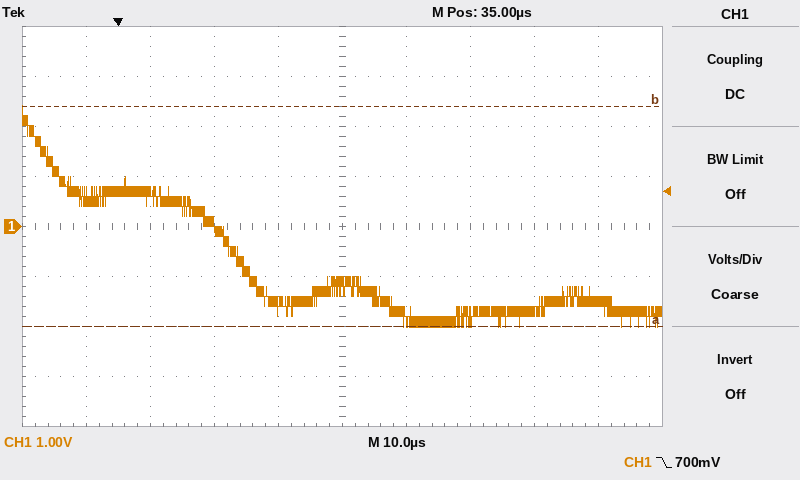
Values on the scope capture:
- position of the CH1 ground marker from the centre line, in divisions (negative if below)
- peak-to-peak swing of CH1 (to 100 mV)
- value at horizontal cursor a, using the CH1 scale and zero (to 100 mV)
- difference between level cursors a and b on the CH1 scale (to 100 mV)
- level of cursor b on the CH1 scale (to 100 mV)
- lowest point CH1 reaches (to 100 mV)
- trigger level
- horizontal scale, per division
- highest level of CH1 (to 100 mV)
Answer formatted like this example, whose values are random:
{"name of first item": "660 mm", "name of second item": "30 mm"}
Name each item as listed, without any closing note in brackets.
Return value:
{"position of the CH1 ground marker from the centre line, in divisions": "0.0 div", "peak-to-peak swing of CH1": "4.4 V", "value at horizontal cursor a, using the CH1 scale and zero": "-2.0 V", "difference between level cursors a and b on the CH1 scale": "4.4 V", "level of cursor b on the CH1 scale": "2.4 V", "lowest point CH1 reaches": "-2.0 V", "trigger level": "700 mV", "horizontal scale, per division": "10 µs", "highest level of CH1": "2.4 V"}
